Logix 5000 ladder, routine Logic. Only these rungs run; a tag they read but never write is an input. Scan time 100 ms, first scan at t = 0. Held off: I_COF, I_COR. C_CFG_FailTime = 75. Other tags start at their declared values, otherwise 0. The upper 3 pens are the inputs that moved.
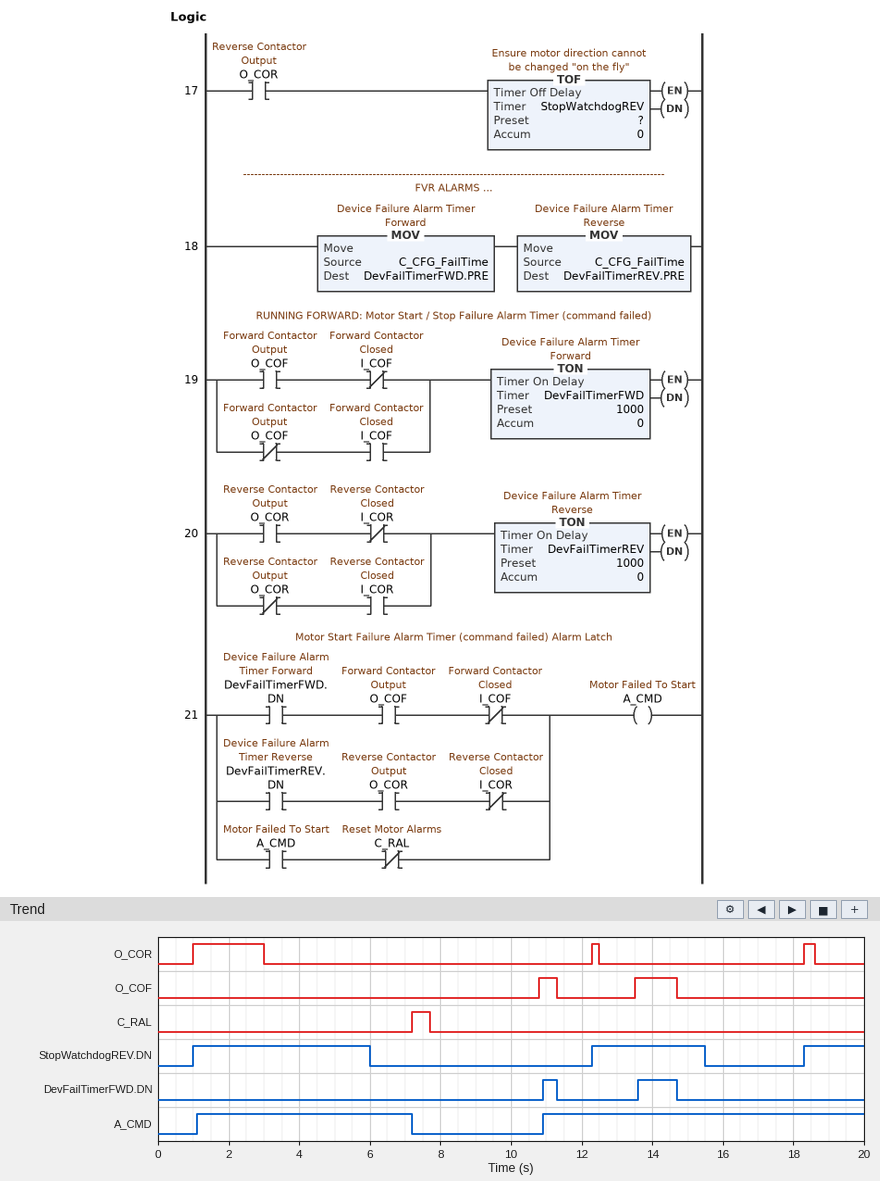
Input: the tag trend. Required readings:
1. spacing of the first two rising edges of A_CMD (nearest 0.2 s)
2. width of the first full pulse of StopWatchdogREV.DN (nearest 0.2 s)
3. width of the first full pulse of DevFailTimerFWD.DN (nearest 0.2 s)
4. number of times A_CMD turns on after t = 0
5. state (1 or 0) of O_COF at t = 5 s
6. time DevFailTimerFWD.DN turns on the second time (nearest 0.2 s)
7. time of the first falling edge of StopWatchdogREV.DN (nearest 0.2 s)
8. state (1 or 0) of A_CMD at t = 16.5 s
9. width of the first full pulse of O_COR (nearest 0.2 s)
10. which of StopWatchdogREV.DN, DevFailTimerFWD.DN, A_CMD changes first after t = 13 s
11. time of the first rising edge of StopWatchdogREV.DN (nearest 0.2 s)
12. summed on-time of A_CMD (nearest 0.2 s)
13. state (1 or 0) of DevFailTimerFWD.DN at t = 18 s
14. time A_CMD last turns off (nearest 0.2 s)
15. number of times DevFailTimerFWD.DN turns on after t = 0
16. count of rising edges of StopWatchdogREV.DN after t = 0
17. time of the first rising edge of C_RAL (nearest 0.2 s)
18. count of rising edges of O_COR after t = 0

9.8 s
5.0 s
0.4 s
2
0
13.6 s
6.0 s
1
2.0 s
DevFailTimerFWD.DN
1.0 s
15.2 s
0
7.2 s
2
3
7.2 s
3
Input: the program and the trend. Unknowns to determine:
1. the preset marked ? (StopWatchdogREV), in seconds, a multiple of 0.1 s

3.0 s
